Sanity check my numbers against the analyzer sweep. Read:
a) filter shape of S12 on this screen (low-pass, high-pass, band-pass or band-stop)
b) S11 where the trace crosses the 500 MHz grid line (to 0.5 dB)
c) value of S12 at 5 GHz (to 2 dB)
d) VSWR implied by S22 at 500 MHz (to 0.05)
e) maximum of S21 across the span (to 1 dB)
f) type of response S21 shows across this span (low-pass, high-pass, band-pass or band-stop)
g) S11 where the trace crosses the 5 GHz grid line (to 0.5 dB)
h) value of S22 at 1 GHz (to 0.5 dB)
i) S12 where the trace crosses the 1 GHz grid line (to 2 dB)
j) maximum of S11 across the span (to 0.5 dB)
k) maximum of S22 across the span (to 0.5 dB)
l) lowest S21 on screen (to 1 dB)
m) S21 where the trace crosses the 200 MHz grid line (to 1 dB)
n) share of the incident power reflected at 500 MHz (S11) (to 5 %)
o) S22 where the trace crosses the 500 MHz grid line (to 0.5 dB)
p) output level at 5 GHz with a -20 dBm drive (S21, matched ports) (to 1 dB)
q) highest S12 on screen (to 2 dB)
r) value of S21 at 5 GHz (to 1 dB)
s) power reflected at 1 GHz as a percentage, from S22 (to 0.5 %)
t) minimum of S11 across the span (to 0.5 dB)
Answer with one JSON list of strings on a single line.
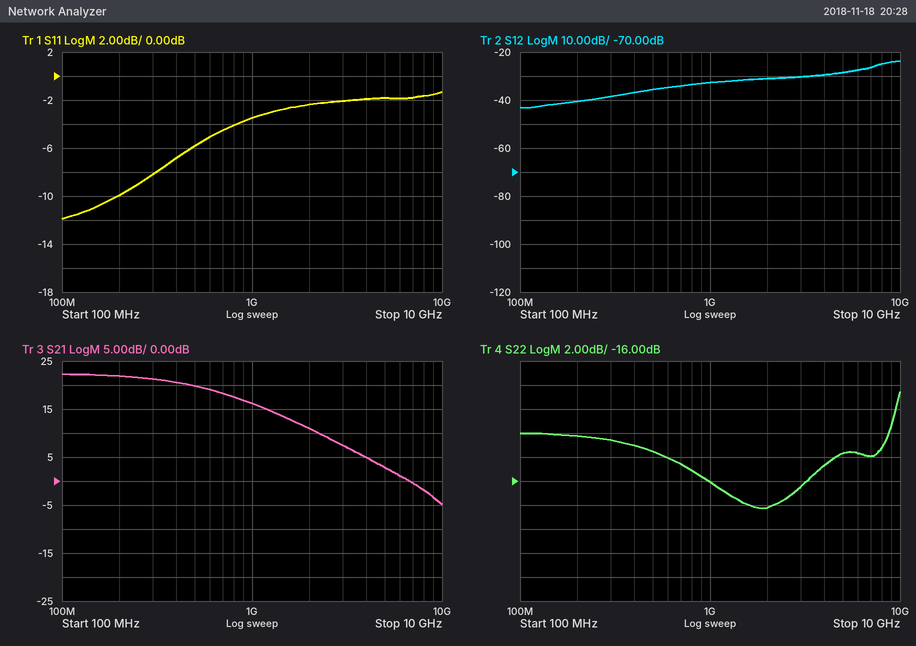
["high-pass", "-6.0 dB", "-28 dB", "1.55", "22 dB", "low-pass", "-2.0 dB", "-16.0 dB", "-32 dB", "-1.5 dB", "-8.5 dB", "-5 dB", "22 dB", "25 %", "-13.5 dB", "-17 dBm", "-24 dB", "3 dB", "2.5 %", "-12.0 dB"]
